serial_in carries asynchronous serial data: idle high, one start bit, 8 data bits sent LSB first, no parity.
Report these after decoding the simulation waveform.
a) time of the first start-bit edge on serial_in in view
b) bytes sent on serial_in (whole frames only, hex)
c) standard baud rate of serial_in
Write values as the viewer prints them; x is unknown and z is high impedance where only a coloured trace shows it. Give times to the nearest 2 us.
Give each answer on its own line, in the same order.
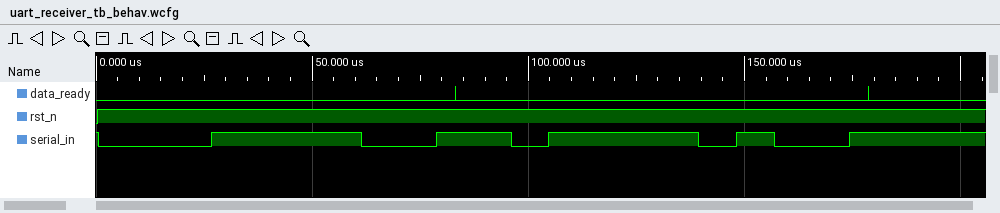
0 us
3C, 2F
115200 baud
